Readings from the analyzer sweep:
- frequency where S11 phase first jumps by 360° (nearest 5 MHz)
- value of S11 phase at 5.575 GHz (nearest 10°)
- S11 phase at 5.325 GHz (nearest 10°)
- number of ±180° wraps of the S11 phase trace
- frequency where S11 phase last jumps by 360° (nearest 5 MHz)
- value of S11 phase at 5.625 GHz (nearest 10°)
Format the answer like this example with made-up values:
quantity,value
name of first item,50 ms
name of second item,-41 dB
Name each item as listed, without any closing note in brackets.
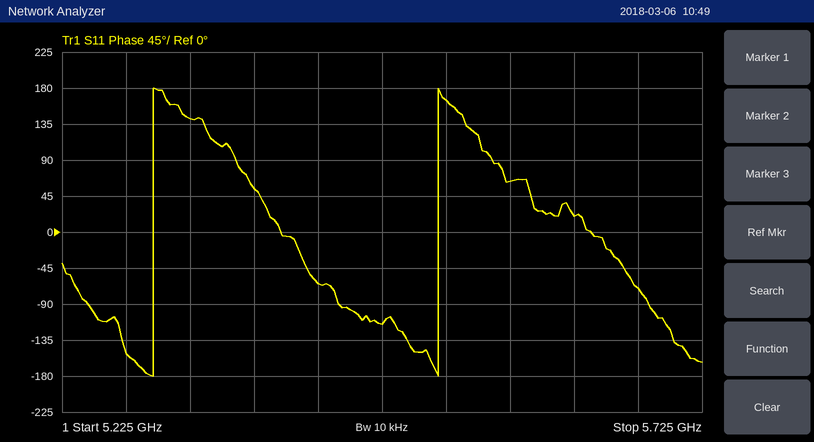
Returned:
quantity,value
frequency where S11 phase first jumps by 360°,5.295 GHz
value of S11 phase at 5.575 GHz,60°
S11 phase at 5.325 GHz,140°
number of ±180° wraps of the S11 phase trace,2
frequency where S11 phase last jumps by 360°,5.520 GHz
value of S11 phase at 5.625 GHz,20°
